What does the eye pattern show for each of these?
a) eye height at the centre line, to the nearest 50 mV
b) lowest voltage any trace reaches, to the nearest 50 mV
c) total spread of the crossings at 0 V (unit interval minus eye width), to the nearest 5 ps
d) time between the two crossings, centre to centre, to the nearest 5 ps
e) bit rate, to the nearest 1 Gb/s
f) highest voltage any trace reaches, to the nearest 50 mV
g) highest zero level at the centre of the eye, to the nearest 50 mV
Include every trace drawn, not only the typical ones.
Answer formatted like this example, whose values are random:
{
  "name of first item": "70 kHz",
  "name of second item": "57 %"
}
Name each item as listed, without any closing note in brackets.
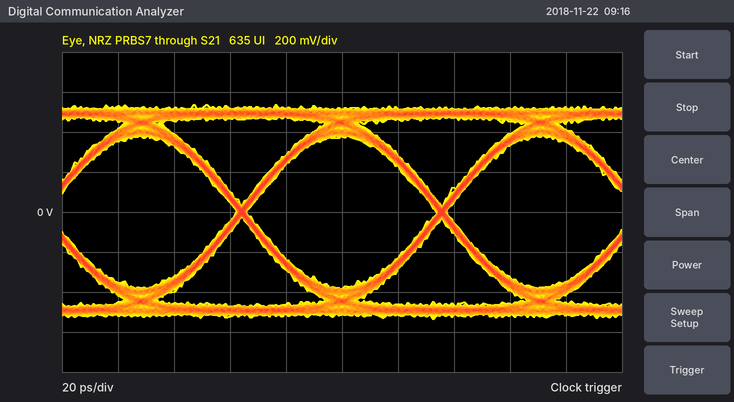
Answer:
{
  "eye height at the centre line, to the nearest 50 mV": "750 mV",
  "lowest voltage any trace reaches, to the nearest 50 mV": "-550 mV",
  "total spread of the crossings at 0 V (unit interval minus eye width), to the nearest 5 ps": "5 ps",
  "time between the two crossings, centre to centre, to the nearest 5 ps": "70 ps",
  "bit rate, to the nearest 1 Gb/s": "14 Gb/s",
  "highest voltage any trace reaches, to the nearest 50 mV": "550 mV",
  "highest zero level at the centre of the eye, to the nearest 50 mV": "-400 mV"
}
